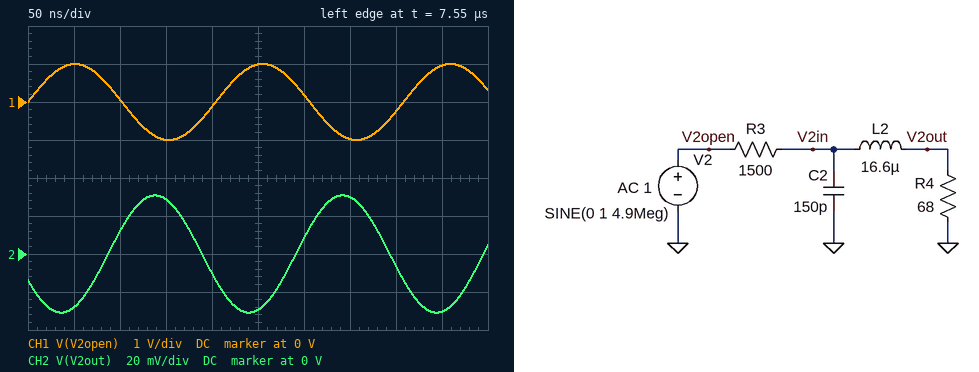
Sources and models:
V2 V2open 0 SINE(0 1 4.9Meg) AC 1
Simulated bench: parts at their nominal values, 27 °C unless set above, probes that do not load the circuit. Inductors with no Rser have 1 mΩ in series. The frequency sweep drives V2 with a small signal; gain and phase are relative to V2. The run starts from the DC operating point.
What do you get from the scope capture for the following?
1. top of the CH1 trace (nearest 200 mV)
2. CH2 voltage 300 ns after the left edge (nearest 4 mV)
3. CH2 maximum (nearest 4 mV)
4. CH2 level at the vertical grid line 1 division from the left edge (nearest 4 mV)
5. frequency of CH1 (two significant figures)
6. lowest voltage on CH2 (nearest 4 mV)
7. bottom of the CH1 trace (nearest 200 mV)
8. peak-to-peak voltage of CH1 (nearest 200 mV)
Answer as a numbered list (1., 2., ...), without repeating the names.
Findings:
1. 1.0 V
2. 8 mV
3. 32 mV
4. -28 mV
5. 4.9 MHz
6. -32 mV
7. -1.0 V
8. 2.0 V
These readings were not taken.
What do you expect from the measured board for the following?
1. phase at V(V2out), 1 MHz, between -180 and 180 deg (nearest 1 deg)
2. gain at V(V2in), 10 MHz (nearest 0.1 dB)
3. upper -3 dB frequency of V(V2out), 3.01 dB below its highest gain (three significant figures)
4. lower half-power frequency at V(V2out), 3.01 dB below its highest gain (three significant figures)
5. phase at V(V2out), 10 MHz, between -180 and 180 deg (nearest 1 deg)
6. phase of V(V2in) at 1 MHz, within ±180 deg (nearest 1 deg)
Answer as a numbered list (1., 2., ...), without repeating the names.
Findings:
1. -8 deg
2. -22.1 dB
3. 3.75 MHz
4. 2.32 MHz
5. -171 deg
6. 49 deg
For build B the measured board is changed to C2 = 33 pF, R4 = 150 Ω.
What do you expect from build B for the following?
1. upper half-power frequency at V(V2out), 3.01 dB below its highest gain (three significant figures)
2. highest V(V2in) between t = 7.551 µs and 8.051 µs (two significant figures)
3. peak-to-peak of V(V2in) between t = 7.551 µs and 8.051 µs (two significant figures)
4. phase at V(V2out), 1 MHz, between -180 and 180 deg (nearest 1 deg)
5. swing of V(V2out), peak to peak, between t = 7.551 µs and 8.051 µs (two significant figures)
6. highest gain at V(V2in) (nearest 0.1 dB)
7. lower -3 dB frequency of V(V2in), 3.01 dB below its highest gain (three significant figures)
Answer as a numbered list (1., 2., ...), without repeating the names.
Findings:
1. 8.45 MHz
2. 470 mV
3. 930 mV
4. -5 deg
5. 260 mV
6. -3.0 dB
7. 5.12 MHz
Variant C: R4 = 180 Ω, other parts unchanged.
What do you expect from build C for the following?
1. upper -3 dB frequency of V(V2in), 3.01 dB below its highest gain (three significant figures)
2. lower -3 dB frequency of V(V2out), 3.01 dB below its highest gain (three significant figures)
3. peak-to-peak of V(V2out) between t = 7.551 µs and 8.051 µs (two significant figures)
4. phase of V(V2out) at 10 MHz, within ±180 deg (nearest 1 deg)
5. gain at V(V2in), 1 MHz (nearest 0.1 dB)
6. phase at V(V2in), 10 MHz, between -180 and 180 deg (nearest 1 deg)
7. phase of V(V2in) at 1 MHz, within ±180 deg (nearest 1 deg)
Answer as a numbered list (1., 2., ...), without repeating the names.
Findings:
1. 4.63 MHz
2. 879 kHz
3. 140 mV
4. -165 deg
5. -17.6 dB
6. -84 deg
7. 17 deg
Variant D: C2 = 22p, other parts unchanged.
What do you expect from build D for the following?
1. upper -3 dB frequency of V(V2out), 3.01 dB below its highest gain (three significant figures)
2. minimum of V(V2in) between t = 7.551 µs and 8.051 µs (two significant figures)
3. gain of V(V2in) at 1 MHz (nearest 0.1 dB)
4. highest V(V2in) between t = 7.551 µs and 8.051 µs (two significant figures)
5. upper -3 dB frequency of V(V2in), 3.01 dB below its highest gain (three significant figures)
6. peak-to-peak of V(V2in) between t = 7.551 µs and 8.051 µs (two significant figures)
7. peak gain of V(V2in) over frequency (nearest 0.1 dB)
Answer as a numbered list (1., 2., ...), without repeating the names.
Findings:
1. 10.1 MHz
2. -430 mV
3. -21.9 dB
4. 430 mV
5. 11.7 MHz
6. 860 mV
7. -1.1 dB
